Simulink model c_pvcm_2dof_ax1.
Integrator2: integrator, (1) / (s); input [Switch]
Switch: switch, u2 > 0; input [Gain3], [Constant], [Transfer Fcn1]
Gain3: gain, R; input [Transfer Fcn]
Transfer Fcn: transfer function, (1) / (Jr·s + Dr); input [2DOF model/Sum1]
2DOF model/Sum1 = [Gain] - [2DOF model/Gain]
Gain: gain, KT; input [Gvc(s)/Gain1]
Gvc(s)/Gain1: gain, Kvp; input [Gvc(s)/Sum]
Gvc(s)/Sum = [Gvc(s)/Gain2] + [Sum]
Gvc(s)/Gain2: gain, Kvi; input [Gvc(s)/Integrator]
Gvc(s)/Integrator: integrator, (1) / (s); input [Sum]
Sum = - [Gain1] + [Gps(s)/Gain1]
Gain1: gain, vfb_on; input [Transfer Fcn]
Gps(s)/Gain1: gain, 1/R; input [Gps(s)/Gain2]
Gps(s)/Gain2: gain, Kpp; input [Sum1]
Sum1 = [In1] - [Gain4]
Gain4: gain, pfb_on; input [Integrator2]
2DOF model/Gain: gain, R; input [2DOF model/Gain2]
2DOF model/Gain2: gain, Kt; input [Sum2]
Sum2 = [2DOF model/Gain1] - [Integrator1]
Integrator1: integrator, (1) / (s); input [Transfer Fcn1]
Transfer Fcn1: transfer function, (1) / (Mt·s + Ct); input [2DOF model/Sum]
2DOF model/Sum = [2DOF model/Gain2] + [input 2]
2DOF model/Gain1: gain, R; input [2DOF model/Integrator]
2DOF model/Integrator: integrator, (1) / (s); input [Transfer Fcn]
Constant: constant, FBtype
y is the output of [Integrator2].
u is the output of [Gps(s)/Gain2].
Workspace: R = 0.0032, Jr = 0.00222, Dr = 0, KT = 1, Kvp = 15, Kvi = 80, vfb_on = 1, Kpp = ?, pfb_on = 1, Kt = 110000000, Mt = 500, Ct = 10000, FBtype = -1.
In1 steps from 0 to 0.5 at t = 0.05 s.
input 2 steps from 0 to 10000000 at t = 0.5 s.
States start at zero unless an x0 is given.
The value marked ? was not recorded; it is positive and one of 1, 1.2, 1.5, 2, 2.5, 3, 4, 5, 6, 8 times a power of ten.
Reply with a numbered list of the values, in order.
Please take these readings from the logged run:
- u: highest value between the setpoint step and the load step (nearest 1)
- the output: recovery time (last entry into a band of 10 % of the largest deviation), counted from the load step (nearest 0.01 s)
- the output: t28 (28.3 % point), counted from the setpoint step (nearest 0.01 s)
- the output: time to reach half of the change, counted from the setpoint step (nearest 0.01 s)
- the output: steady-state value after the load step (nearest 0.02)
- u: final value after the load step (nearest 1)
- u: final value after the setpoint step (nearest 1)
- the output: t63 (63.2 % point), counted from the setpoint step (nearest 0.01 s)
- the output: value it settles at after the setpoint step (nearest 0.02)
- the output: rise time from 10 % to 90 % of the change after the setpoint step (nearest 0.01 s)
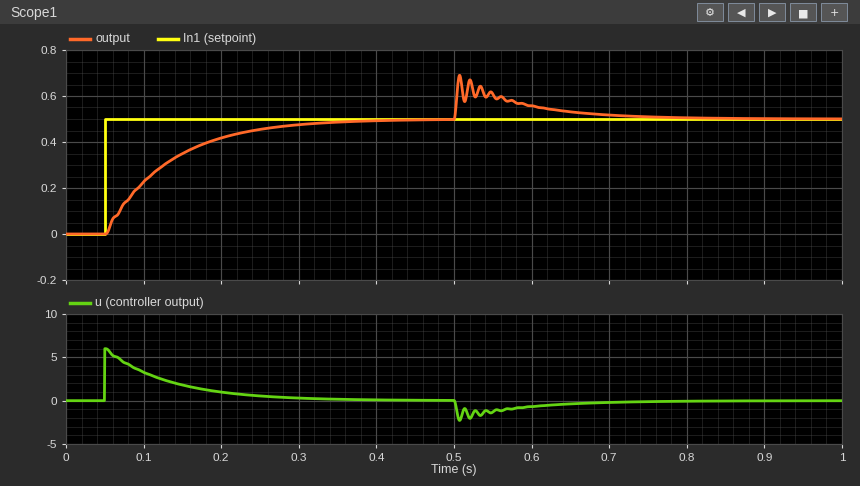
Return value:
1. 6
2. 0.19 s
3. 0.03 s
4. 0.06 s
5. 0.50
6. 0
7. 0
8. 0.08 s
9. 0.50
10. 0.18 s
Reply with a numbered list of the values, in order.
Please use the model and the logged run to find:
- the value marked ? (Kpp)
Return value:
1. 12
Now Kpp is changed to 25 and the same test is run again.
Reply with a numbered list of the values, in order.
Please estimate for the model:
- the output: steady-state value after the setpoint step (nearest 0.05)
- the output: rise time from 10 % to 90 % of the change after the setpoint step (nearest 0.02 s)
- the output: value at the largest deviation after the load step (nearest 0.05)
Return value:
1. 0.50
2. 0.08 s
3. 0.70
